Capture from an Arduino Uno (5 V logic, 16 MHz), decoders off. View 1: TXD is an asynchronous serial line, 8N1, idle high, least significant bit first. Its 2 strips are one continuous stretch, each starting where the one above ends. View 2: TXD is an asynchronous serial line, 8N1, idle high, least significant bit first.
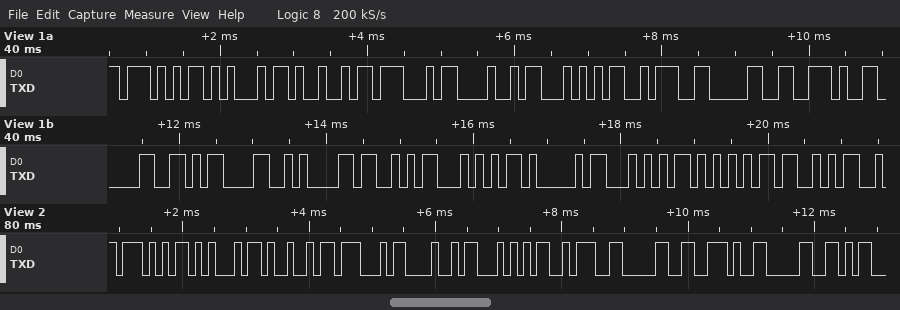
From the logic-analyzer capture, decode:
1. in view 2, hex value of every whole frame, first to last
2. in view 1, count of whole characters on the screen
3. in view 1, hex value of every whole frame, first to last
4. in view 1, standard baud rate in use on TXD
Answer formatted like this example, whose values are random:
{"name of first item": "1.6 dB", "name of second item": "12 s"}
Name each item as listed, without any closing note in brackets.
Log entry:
{"in view 2, hex value of every whole frame, first to last": "57 45 49 47 48 54 3A 30 2E 30", "in view 1, count of whole characters on the screen": "18", "in view 1, hex value of every whole frame, first to last": "57 45 49 47 48 54 3A 30 2E 30 0D 0A 53 54 41 54 55 53", "in view 1, standard baud rate in use on TXD": "9600 baud"}
